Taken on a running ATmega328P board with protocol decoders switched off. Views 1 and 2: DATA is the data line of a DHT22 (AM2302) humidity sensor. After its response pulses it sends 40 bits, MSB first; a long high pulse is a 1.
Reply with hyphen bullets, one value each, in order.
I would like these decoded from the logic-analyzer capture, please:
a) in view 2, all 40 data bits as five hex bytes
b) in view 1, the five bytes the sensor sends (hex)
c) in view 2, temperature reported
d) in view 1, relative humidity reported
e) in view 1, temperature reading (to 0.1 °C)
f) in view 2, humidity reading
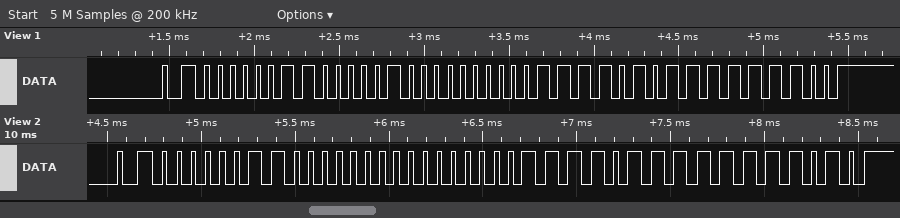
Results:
- 03 00 00 F7 FA
- 03 04 00 F5 FC
- 24.7 °C
- 77.2 %
- 24.5 °C
- 76.8 %
